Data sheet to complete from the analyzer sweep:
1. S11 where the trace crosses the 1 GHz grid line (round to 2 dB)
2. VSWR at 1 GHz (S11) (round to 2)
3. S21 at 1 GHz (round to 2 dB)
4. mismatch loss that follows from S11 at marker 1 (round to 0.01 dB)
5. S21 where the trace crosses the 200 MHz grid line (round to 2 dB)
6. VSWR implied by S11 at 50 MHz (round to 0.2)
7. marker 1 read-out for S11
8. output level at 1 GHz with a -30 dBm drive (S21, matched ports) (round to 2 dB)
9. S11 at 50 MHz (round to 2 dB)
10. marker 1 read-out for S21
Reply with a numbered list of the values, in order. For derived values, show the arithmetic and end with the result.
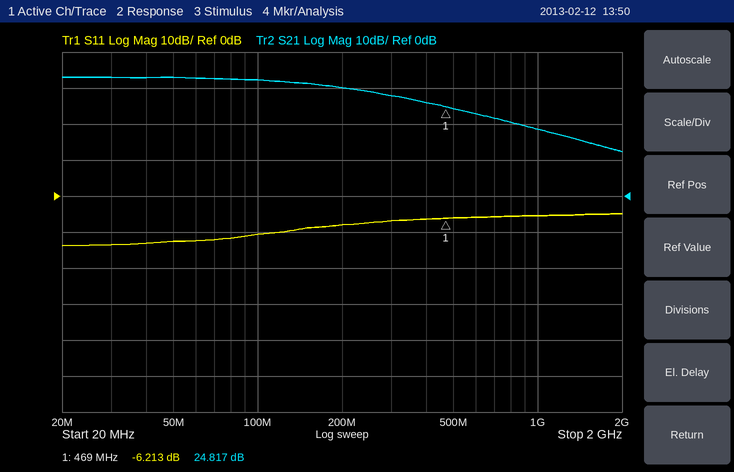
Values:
1. -6 dB
2. |Γ| = 10^(-6/20) = 0.5012; VSWR = (1 + 0.5012)/(1 − 0.5012) ≈ 3.01, so 4 to the nearest 2
3. 18 dB
4. −10 log10(1 − 10^(-6.213/10)) ≈ 1.19 dB
5. 30 dB
6. |Γ| = 10^(-12/20) = 0.2512; VSWR = (1 + 0.2512)/(1 − 0.2512) ≈ 1.67, so 1.6 to the nearest 0.2
7. -6.213 dB
8. -30 dBm + (18 dB) = -12 dBm
9. -12 dB
10. 24.817 dB
